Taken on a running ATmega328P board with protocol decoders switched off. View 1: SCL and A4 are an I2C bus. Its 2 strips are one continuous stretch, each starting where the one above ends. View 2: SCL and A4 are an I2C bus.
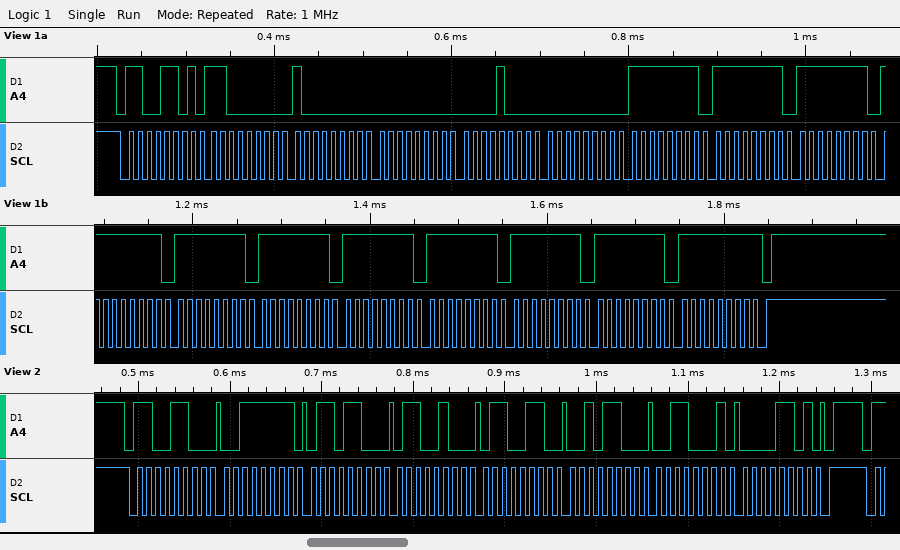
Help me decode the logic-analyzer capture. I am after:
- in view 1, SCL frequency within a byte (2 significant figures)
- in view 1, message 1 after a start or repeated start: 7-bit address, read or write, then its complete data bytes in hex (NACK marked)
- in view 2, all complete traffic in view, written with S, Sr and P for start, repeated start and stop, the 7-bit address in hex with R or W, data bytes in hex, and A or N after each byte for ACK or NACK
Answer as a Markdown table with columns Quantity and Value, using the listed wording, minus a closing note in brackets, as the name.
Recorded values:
| Quantity | Value |
|---|---|
| in view 1, SCL frequency within a byte | 100 kHz |
| in view 1, message 1 after a start or repeated start: 7-bit address, read or write, then its complete data bytes in hex | 0x66 read: C0 80 00 08 00 FF FF FF FF FF FF FF FF FF FF FF NACK |
| in view 2, all complete traffic in view, written with S, Sr and P for start, repeated start and stop, the 7-bit address in hex with R or W, data bytes in hex, and A or N after each byte for ACK or NACK | S 66W A 3F A 6C A 64 A 66 A 2C A 31 A 0D A P |
